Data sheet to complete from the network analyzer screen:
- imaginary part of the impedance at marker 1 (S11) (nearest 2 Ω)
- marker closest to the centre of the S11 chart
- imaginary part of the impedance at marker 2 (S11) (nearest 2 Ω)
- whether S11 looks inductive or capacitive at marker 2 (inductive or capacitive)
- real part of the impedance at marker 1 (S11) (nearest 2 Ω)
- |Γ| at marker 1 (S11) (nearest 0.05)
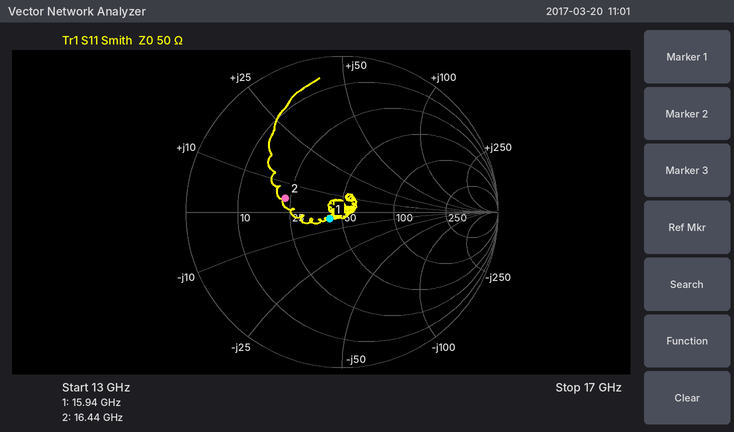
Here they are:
-4 Ω
marker 1
+4 Ω
inductive
42 Ω
0.10
